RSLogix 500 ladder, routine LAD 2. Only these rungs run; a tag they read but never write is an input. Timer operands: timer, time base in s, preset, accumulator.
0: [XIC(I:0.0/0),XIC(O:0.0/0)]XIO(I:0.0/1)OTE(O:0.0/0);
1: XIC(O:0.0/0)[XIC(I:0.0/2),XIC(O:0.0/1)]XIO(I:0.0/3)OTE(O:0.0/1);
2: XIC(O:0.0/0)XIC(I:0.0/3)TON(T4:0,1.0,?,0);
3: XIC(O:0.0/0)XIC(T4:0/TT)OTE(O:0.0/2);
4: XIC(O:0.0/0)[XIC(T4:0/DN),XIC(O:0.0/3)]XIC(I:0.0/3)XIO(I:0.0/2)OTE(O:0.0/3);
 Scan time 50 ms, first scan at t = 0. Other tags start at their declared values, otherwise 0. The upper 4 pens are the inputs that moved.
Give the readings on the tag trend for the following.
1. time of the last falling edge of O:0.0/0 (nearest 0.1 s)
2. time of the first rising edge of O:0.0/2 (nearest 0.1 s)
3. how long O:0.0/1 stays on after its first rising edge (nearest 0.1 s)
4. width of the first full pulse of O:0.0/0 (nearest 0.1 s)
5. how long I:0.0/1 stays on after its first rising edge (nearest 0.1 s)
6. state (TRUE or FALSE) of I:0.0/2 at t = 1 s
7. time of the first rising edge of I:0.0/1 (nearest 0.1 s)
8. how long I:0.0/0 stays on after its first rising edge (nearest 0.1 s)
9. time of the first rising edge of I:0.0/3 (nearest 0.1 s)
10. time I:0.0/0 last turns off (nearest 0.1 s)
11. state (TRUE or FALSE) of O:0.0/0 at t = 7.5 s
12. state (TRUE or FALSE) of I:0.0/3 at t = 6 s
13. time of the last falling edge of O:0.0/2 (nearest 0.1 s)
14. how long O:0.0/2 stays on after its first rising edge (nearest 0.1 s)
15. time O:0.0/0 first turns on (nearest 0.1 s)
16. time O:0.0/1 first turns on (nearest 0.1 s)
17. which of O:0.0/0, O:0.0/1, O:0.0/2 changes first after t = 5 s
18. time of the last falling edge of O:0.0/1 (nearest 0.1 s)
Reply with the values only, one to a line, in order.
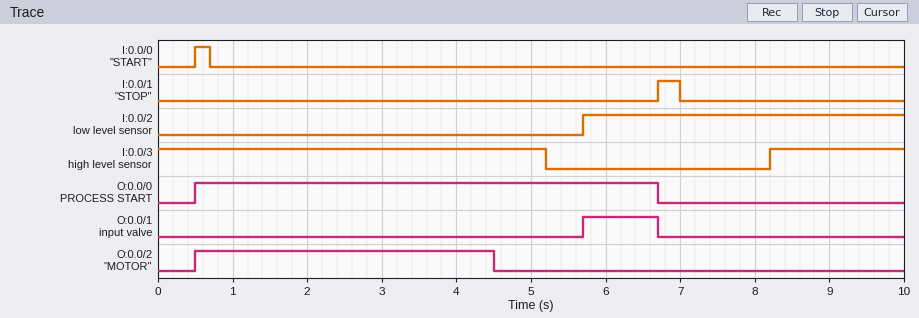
6.7 s
0.5 s
1.0 s
6.2 s
0.3 s
FALSE
6.7 s
0.2 s
8.2 s
0.7 s
FALSE
FALSE
4.5 s
4.0 s
0.5 s
5.7 s
O:0.0/1
6.7 s
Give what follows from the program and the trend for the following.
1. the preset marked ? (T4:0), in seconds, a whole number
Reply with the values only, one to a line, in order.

4 s
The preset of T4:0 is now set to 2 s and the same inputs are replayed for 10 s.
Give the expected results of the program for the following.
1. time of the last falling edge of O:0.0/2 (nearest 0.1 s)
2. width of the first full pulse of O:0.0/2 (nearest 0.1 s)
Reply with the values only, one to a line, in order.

2.5 s
2.0 s
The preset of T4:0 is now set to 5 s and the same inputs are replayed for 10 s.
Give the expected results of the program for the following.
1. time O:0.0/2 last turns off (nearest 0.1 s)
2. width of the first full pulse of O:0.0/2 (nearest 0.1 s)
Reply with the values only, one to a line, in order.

5.2 s
4.7 s
